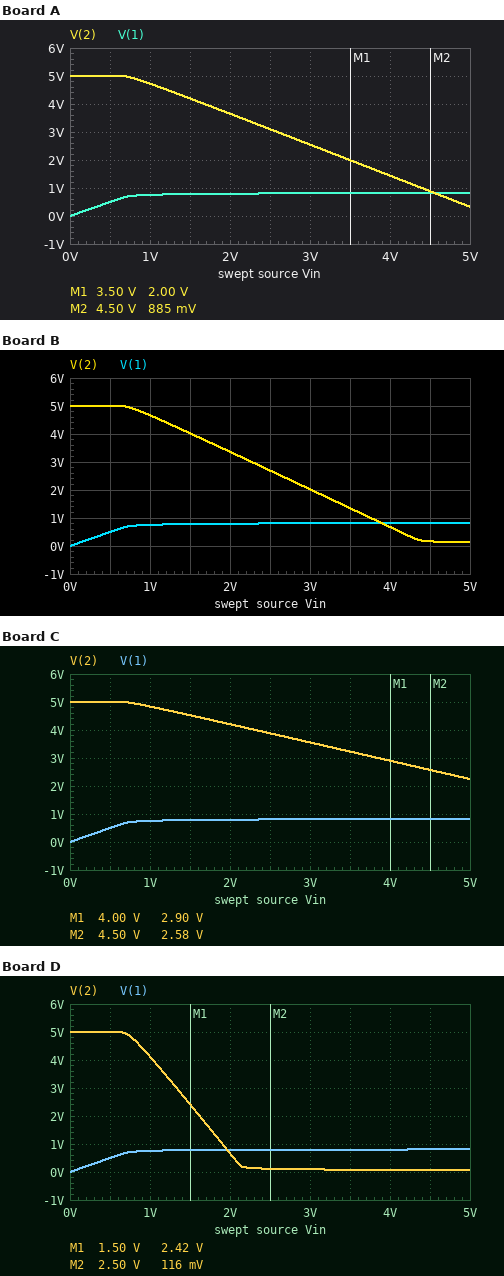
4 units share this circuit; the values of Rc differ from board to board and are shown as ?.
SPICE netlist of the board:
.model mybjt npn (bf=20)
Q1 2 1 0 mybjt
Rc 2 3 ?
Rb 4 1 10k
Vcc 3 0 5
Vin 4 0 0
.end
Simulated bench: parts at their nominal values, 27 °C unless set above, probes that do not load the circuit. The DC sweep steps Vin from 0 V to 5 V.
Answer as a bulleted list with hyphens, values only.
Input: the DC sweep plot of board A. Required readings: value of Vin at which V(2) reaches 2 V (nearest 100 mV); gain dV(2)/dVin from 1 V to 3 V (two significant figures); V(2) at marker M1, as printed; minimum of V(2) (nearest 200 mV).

- 3.5 V
- -1.1 V/V
- 2.00 V
- 400 mV
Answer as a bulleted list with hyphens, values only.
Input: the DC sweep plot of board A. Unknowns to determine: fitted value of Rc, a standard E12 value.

- 560 Ω
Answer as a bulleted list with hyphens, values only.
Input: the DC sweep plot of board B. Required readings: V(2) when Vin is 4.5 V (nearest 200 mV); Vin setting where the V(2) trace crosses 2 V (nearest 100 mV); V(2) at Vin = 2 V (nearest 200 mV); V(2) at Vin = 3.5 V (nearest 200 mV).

- 200 mV
- 3.0 V
- 3.4 V
- 1.4 V
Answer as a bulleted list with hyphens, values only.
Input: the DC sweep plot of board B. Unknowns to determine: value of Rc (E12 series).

- 680 Ω
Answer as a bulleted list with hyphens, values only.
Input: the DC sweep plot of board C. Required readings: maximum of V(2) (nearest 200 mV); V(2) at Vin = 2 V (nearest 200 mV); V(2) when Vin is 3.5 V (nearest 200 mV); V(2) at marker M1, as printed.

- 5.0 V
- 4.2 V
- 3.2 V
- 2.90 V
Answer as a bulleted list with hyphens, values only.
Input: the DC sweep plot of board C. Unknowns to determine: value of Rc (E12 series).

- 330 Ω
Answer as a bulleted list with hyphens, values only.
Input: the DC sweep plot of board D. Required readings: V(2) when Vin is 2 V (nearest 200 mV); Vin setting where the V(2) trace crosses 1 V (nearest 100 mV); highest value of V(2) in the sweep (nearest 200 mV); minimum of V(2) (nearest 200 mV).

- 600 mV
- 1.9 V
- 5.0 V
- 0 V
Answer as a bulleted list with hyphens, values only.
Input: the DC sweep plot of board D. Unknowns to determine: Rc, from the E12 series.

- 1.8 kΩ
